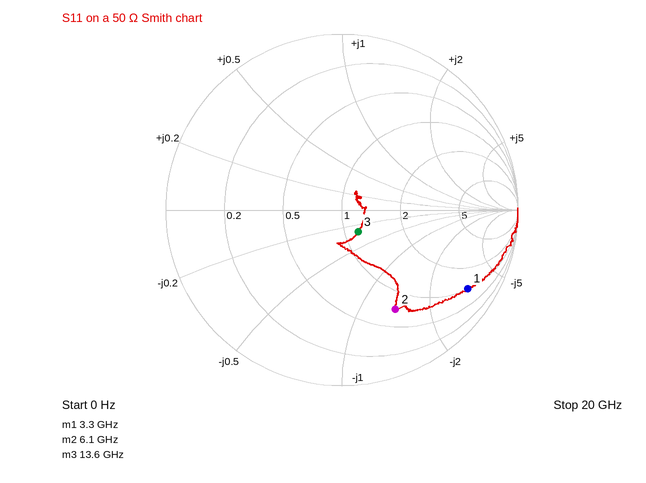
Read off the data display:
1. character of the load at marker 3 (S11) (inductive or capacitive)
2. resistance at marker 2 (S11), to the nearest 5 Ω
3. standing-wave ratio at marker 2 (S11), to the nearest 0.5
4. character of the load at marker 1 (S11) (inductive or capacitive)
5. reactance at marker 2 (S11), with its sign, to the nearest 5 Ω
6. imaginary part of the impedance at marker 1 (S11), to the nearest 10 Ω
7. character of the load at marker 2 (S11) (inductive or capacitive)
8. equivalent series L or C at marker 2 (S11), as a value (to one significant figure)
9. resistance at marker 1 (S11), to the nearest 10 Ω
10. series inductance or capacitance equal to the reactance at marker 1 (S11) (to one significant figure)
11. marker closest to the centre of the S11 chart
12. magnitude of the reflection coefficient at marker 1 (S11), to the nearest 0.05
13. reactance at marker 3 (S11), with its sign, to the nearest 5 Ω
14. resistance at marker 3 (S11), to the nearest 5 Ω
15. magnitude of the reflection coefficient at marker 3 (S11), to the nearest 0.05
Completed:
capacitive
35 Ω
4.5
capacitive
-70 Ω
-160 Ω
capacitive
400 fF
50 Ω
300 fF
marker 3
0.85
-15 Ω
60 Ω
0.15
